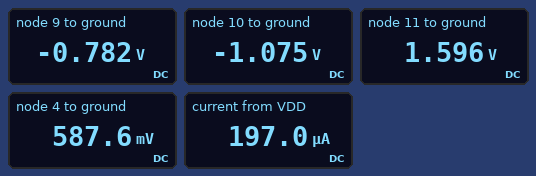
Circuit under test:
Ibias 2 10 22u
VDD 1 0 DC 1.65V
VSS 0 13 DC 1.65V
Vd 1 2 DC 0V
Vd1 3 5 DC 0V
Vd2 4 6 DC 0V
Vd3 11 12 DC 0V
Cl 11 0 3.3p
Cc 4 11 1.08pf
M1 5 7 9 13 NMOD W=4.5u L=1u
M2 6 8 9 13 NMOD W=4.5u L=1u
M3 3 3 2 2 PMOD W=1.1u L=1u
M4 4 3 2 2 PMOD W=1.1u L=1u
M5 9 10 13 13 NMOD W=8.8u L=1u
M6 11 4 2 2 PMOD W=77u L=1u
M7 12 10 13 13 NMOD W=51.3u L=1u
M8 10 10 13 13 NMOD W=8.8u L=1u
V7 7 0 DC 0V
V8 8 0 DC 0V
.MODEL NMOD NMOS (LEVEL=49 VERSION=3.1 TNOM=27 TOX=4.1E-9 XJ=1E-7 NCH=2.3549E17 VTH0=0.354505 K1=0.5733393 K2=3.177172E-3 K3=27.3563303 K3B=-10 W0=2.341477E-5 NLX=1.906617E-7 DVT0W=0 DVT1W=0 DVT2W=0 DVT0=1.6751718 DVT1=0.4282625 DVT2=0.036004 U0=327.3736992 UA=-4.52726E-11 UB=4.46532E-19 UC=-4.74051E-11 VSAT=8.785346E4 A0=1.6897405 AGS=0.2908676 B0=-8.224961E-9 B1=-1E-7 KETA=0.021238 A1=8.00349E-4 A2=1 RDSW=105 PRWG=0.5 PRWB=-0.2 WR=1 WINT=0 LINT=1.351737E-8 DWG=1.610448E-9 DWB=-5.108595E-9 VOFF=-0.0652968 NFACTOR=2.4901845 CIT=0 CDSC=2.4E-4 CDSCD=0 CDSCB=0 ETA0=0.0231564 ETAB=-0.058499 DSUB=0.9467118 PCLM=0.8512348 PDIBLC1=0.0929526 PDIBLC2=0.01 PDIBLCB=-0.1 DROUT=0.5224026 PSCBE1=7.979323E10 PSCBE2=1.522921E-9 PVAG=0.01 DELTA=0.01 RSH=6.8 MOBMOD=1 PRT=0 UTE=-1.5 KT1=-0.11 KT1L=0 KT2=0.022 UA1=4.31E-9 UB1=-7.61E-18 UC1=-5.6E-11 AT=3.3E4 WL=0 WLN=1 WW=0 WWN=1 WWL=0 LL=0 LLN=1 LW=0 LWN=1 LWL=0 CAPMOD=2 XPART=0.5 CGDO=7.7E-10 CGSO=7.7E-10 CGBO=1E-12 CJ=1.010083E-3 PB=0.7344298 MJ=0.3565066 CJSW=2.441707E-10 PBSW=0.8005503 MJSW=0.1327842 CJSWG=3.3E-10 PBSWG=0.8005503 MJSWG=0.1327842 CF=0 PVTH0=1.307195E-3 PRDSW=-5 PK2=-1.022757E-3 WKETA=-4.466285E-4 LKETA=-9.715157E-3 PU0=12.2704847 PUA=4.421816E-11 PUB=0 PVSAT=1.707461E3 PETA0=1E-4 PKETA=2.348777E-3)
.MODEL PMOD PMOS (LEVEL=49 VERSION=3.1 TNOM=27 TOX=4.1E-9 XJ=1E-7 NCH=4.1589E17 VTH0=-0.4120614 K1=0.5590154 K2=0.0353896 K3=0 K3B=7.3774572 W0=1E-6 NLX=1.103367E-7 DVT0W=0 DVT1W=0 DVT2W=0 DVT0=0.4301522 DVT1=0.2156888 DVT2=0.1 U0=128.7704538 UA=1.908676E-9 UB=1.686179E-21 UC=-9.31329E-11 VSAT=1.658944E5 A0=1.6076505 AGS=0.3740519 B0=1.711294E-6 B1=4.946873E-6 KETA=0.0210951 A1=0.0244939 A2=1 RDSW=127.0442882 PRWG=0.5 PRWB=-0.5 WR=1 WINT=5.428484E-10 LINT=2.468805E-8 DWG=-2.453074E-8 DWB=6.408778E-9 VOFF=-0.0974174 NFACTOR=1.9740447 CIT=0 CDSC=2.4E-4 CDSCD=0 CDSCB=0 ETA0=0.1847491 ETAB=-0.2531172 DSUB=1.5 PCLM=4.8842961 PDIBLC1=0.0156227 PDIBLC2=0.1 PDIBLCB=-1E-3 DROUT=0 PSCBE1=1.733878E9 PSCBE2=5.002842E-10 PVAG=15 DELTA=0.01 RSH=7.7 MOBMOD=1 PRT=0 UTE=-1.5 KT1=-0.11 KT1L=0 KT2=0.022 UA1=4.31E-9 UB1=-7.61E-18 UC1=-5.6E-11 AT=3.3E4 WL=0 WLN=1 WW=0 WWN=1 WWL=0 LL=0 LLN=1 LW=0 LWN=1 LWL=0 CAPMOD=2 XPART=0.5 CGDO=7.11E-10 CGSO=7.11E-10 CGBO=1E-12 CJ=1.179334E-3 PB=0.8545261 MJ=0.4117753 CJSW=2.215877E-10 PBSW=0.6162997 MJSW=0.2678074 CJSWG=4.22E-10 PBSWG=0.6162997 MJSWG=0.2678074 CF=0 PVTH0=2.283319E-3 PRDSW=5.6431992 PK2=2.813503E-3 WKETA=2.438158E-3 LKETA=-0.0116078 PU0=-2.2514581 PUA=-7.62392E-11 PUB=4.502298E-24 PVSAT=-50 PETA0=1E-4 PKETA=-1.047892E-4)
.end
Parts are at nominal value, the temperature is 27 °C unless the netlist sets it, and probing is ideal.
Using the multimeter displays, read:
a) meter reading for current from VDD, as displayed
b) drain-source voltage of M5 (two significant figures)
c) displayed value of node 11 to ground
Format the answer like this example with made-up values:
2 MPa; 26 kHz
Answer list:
197.0 µA; 870 mV; 1.596 V
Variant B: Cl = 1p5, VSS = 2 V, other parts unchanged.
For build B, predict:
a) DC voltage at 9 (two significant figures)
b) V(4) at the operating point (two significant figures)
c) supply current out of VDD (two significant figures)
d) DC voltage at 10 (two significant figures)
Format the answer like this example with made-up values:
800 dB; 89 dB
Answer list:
-840 mV; 580 mV; 200 µA; -1.4 V
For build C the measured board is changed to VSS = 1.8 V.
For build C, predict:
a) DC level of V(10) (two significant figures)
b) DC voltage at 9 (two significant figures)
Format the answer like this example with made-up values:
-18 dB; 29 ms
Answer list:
-1.2 V; -810 mV
